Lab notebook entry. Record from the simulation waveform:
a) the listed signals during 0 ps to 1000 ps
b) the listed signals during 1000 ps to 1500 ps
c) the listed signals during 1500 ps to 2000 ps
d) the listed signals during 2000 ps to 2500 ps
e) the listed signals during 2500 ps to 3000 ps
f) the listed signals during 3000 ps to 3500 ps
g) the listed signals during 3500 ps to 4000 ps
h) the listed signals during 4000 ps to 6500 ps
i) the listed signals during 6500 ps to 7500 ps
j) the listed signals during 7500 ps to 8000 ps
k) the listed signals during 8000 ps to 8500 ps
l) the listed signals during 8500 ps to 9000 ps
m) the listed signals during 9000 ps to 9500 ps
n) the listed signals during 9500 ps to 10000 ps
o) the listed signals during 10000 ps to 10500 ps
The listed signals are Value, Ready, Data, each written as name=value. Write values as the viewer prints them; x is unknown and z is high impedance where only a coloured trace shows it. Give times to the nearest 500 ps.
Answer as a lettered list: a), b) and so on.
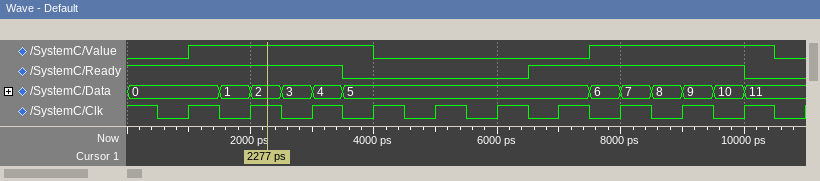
a) Value=0, Ready=1, Data=0
b) Value=1, Ready=1, Data=0
c) Value=1, Ready=1, Data=1
d) Value=1, Ready=1, Data=2
e) Value=1, Ready=1, Data=3
f) Value=1, Ready=1, Data=4
g) Value=1, Ready=0, Data=5
h) Value=0, Ready=0, Data=5
i) Value=0, Ready=1, Data=5
j) Value=1, Ready=1, Data=6
k) Value=1, Ready=1, Data=7
l) Value=1, Ready=1, Data=8
m) Value=1, Ready=1, Data=9
n) Value=1, Ready=1, Data=10
o) Value=1, Ready=0, Data=11
